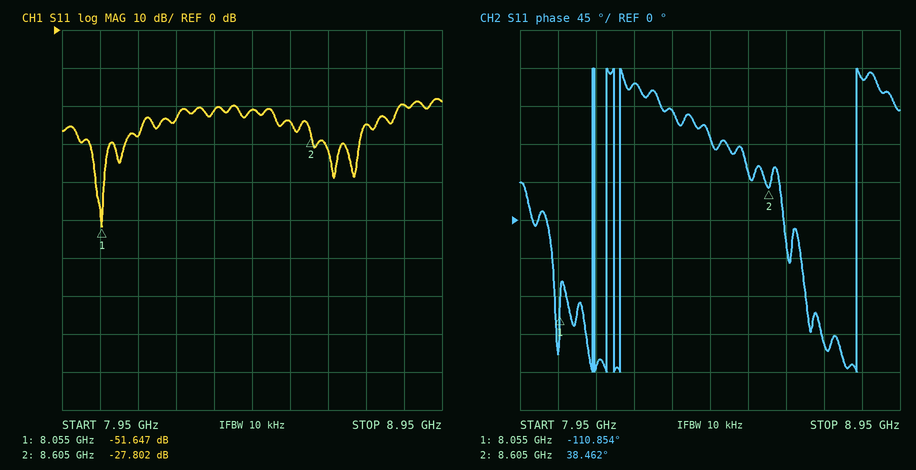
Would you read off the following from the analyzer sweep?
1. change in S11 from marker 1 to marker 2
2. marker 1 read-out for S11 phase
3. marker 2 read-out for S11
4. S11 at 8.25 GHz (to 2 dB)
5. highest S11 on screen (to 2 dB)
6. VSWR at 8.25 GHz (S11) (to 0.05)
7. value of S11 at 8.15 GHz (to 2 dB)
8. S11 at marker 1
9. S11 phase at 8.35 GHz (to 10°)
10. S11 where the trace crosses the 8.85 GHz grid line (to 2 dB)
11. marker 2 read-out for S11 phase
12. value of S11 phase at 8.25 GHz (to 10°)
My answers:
23.845 dB
-110.854°
-27.802 dB
-24 dB
-18 dB
1.15
-28 dB
-51.647 dB
130°
-20 dB
38.462°
160°
